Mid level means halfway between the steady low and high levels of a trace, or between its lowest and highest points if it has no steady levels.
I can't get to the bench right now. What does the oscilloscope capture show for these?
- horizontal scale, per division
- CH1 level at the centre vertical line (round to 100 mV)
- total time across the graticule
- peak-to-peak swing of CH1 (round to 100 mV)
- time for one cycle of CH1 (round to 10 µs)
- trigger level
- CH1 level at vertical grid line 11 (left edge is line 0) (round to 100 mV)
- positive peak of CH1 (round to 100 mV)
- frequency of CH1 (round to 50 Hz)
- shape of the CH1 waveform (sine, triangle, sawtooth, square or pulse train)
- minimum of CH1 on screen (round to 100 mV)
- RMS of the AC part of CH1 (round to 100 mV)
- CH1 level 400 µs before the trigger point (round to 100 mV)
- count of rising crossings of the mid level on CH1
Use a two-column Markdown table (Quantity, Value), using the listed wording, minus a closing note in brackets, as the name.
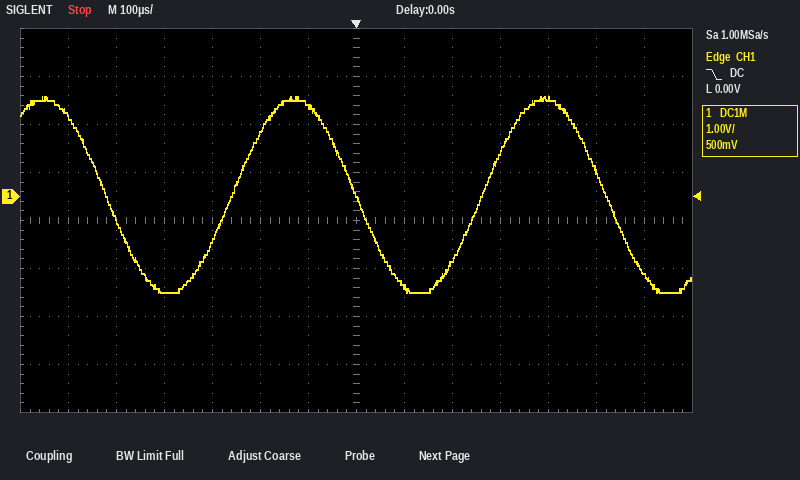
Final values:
| Quantity | Value |
|---|---|
| horizontal scale, per division | 100 µs |
| CH1 level at the centre vertical line | 0.0 V |
| total time across the graticule | 1.4 ms |
| peak-to-peak swing of CH1 | 4.1 V |
| time for one cycle of CH1 | 520 µs |
| trigger level | 0.00 V |
| CH1 level at vertical grid line 11 (left edge is line 0) | 2.0 V |
| positive peak of CH1 | 2.1 V |
| frequency of CH1 | 1.90 kHz |
| shape of the CH1 waveform | sine |
| minimum of CH1 on screen | -2.0 V |
| RMS of the AC part of CH1 | 1.4 V |
| CH1 level 400 µs before the trigger point | -2.0 V |
| count of rising crossings of the mid level on CH1 | 2 |
